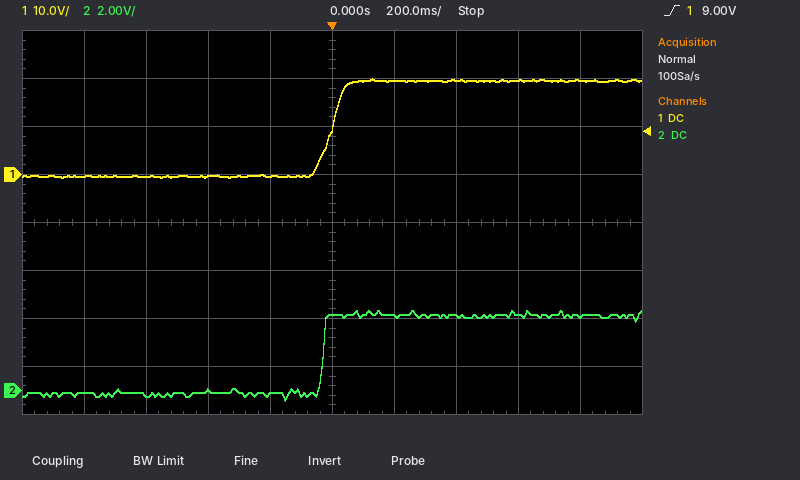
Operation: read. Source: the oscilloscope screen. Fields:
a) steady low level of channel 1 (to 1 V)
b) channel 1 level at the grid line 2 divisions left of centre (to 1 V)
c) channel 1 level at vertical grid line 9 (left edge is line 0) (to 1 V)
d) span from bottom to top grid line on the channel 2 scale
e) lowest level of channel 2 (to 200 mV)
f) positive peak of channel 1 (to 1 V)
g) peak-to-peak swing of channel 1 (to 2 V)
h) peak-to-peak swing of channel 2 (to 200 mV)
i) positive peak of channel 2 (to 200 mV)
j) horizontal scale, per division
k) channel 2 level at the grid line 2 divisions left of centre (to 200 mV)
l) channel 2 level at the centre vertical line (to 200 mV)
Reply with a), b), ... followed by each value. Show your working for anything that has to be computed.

a) 0 V
b) 0 V
c) 20 V
d) 16 V
e) -400 mV
f) 20 V
g) 20 V
h) 3.4 V − (-400 mV) = 3.8 V
i) 3.4 V
j) 200 ms
k) 0.0 V
l) 3.2 V
